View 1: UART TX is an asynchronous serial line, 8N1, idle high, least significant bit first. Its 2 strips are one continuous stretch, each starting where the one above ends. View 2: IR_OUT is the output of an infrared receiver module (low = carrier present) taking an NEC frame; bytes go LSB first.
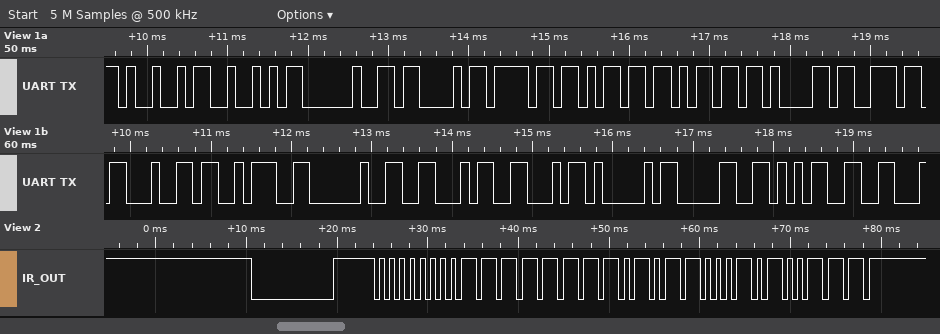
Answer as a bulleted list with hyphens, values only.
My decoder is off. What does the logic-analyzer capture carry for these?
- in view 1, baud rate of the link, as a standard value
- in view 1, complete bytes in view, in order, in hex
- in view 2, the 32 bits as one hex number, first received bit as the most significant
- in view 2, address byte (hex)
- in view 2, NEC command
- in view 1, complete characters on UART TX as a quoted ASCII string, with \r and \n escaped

- 9600 baud
- 49 52 20 43 6F 6D 6D 61 6E 64 3A 20 46 46 41 30 35
- 0x00FF58A7
- 0x00
- 0x1A
- "IR Command: FFA05"
